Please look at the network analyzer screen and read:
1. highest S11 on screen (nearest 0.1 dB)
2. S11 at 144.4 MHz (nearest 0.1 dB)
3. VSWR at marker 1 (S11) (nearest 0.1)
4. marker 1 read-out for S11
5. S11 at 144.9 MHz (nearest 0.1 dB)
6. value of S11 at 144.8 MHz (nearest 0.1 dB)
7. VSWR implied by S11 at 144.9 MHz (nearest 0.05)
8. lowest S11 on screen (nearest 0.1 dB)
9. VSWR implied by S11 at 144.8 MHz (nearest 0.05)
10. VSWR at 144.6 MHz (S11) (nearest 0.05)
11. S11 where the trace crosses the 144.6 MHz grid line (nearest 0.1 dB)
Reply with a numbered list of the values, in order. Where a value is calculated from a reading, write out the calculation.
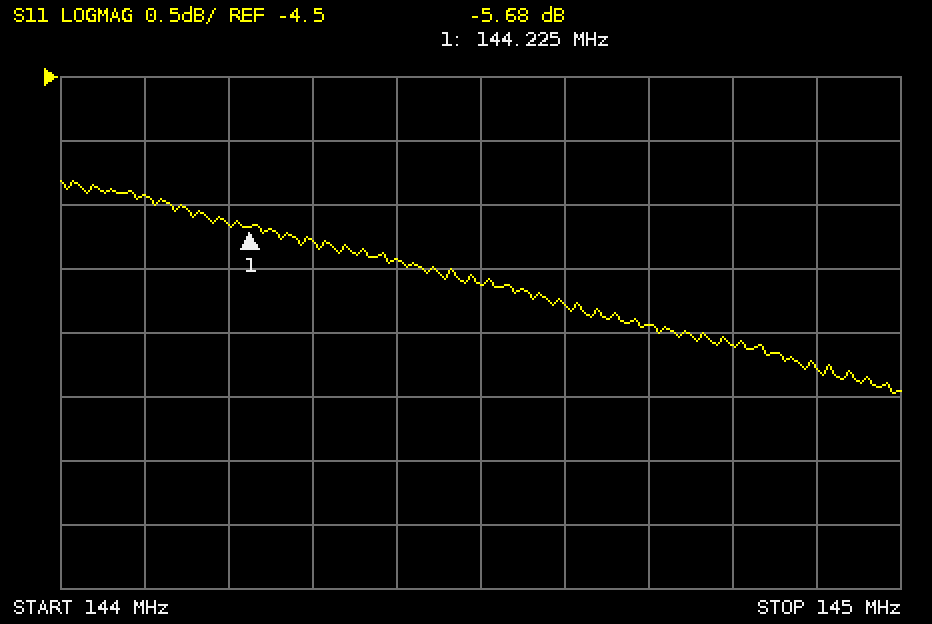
1. -5.3 dB
2. -5.9 dB
3. (1 + 0.5200)/(1 − 0.5200) ≈ 3.2
4. -5.68 dB
5. -6.8 dB
6. -6.6 dB
7. |Γ| = 10^(-6.8/20) = 0.4571; VSWR = (1 + 0.4571)/(1 − 0.4571) ≈ 2.68, so 2.70 to the nearest 0.05
8. -7.0 dB
9. |Γ| = 10^(-6.6/20) = 0.4677; VSWR = (1 + 0.4677)/(1 − 0.4677) ≈ 2.76, so 2.75 to the nearest 0.05
10. |Γ| = 10^(-6.3/20) = 0.4842; VSWR = (1 + 0.4842)/(1 − 0.4842) ≈ 2.88, so 2.90 to the nearest 0.05
11. -6.3 dB
